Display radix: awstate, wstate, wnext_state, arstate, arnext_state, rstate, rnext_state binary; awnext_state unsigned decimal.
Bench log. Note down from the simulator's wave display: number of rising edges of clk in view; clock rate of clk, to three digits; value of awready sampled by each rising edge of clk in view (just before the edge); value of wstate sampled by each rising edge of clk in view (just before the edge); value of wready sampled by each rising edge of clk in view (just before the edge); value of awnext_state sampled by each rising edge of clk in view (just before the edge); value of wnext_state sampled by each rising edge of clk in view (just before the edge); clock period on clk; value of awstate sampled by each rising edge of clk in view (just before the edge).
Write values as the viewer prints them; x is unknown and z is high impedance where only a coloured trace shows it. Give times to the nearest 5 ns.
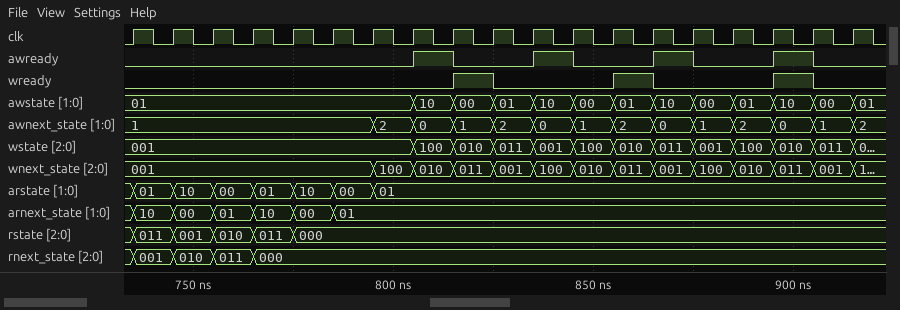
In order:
19
100 MHz
0 0 0 0 0 0 0 0 1 0 0 1 0 0 1 0 0 1 0
001, 001, 001, 001, 001, 001, 001, 001, 100, 010, 011, 001, 100, 010, 011, 001, 100, 010, 011
0 0 0 0 0 0 0 0 0 1 0 0 0 1 0 0 0 1 0
1, 1, 1, 1, 1, 1, 1, 2, 0, 1, 2, 0, 1, 2, 0, 1, 2, 0, 1
001, 001, 001, 001, 001, 001, 001, 100, 010, 011, 001, 100, 010, 011, 001, 100, 010, 011, 001
10 ns
01, 01, 01, 01, 01, 01, 01, 01, 10, 00, 01, 10, 00, 01, 10, 00, 01, 10, 00
